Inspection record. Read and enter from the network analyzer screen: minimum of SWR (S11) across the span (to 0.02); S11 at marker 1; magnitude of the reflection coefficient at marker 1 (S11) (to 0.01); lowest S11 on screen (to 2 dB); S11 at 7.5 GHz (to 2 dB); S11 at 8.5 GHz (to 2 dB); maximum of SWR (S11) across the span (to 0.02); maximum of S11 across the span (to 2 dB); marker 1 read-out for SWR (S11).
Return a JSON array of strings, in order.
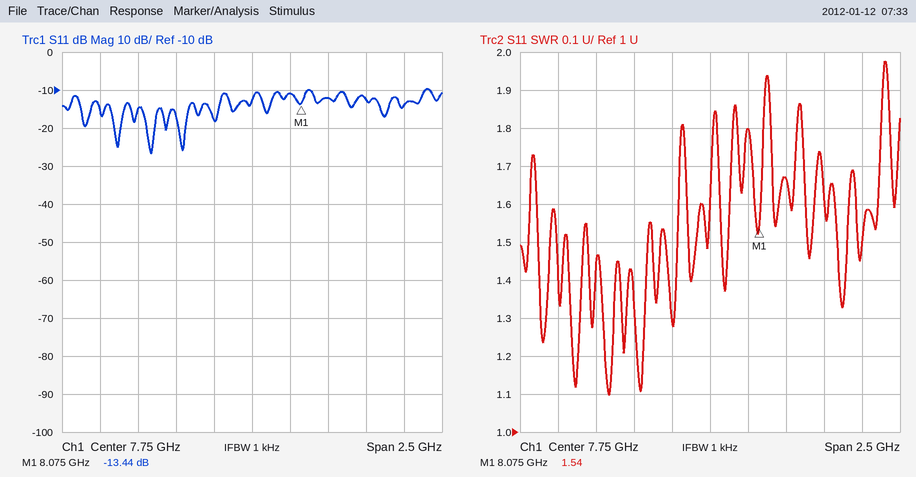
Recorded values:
["1.10", "-13.44 dB", "0.21", "-26 dB", "-18 dB", "-12 dB", "1.98", "-10 dB", "1.54"]
